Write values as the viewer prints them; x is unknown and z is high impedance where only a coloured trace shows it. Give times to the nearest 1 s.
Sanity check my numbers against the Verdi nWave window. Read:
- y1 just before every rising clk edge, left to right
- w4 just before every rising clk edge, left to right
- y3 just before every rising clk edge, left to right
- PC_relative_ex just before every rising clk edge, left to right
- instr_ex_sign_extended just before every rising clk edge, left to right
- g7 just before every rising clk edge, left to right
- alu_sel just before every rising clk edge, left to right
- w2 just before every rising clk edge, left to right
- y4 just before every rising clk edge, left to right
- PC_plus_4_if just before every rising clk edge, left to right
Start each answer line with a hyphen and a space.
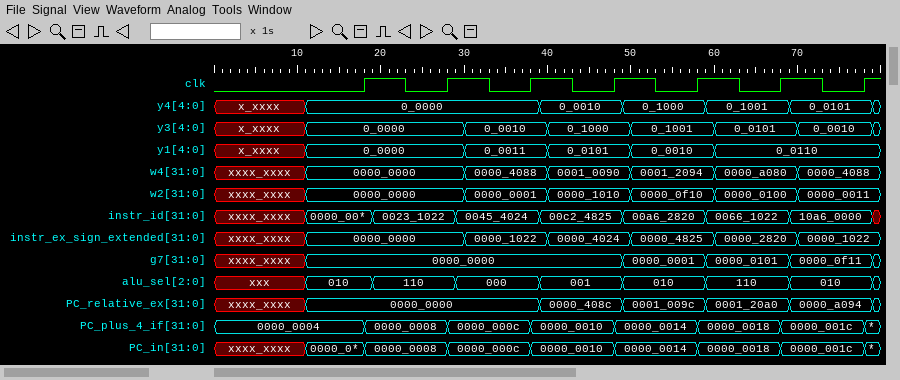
- 0_0000, 0_0000, 0_0011, 0_0101, 0_0010, 0_0110, 0_0110
- 0000_0000, 0000_0000, 0000_4088, 0001_0090, 0001_2094, 0000_a080, 0000_4088
- 0_0000, 0_0000, 0_0010, 0_1000, 0_1001, 0_0101, 0_0010
- 0000_0000, 0000_0000, 0000_0000, 0000_408c, 0001_009c, 0001_20a0, 0000_a094
- 0000_0000, 0000_0000, 0000_1022, 0000_4024, 0000_4825, 0000_2820, 0000_1022
- 0000_0000, 0000_0000, 0000_0000, 0000_0000, 0000_0001, 0000_0101, 0000_0f11
- 010, 110, 000, 001, 010, 110, 010
- 0000_0000, 0000_0000, 0000_0001, 0000_1010, 0000_0f10, 0000_0100, 0000_0011
- 0_0000, 0_0000, 0_0000, 0_0010, 0_1000, 0_1001, 0_0101
- 0000_0004, 0000_0008, 0000_000c, 0000_0010, 0000_0014, 0000_0018, 0000_001c
